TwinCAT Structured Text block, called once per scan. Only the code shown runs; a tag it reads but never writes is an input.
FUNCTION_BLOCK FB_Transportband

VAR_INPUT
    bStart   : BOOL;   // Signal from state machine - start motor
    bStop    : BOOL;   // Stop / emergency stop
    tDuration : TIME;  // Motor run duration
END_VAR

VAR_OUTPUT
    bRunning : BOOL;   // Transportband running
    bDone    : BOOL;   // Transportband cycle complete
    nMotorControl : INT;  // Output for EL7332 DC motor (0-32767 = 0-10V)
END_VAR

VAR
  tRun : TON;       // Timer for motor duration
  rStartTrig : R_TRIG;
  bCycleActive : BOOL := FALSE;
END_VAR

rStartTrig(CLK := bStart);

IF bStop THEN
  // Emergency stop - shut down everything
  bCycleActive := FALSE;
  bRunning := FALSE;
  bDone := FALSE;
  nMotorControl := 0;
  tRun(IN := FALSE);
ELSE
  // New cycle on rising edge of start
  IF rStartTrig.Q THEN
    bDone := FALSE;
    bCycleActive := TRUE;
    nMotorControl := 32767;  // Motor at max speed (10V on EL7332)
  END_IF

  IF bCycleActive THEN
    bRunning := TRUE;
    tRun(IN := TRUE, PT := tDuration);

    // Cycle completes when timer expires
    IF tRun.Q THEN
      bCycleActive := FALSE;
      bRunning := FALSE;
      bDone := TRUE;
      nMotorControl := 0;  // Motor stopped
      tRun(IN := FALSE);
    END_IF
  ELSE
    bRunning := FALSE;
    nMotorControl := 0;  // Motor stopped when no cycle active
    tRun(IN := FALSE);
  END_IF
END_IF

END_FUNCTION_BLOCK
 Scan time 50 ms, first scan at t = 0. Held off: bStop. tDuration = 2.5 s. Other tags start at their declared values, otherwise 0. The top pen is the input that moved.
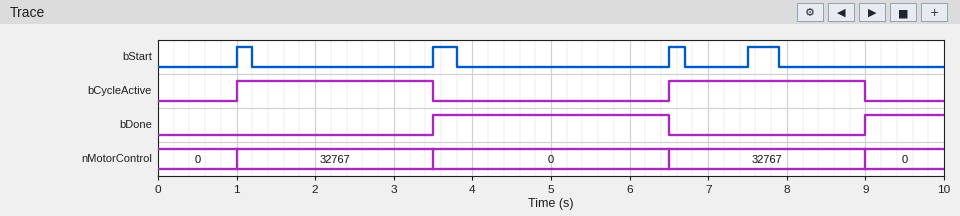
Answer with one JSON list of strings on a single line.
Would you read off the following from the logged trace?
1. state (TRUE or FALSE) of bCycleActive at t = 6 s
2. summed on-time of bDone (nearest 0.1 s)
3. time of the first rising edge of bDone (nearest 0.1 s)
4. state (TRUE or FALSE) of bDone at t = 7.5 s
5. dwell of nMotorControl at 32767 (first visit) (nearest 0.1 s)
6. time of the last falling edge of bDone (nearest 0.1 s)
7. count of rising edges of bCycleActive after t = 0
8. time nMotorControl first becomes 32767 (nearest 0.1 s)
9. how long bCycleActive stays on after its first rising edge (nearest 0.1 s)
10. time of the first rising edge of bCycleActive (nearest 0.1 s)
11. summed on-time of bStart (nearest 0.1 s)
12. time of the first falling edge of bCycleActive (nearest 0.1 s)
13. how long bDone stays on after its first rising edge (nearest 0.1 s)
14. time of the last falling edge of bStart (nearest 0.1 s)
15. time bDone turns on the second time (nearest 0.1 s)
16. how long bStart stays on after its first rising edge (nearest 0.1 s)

["FALSE", "4.0 s", "3.5 s", "FALSE", "2.5 s", "6.5 s", "2", "1.0 s", "2.5 s", "1.0 s", "1.1 s", "3.5 s", "3.0 s", "7.9 s", "9.0 s", "0.2 s"]
